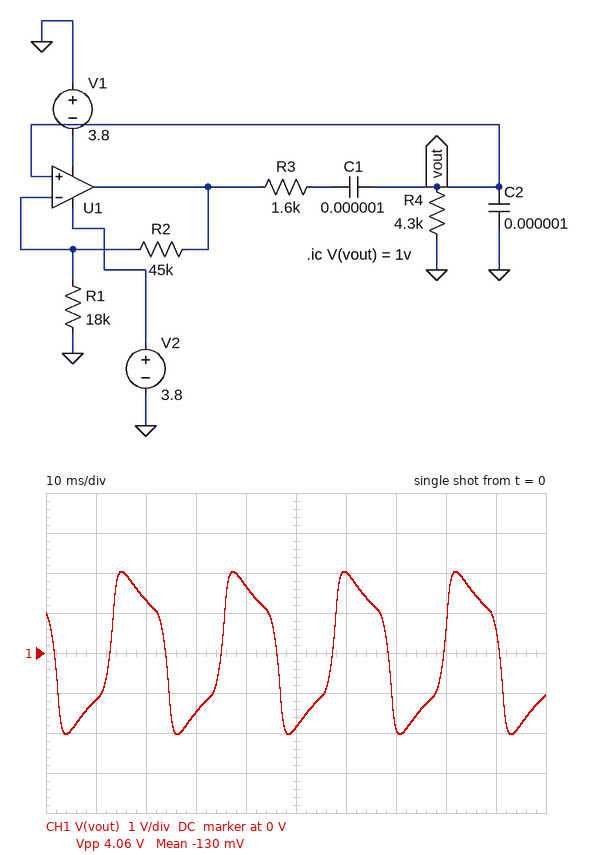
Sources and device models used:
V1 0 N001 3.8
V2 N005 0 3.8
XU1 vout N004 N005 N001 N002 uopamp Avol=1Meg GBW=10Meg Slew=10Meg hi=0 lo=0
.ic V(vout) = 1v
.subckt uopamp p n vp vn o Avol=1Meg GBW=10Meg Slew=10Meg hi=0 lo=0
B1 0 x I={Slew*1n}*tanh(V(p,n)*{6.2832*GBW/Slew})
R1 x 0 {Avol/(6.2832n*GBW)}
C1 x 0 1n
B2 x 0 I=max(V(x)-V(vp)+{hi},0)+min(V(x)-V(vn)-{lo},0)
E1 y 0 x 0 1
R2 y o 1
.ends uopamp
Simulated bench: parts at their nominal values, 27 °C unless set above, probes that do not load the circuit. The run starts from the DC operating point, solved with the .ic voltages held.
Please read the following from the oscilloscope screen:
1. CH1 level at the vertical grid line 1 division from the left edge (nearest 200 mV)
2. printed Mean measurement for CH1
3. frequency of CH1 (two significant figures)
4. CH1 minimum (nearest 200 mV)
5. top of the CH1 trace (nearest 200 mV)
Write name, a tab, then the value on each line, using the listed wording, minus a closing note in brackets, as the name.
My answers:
CH1 level at the vertical grid line 1 division from the left edge	-1.2 V
printed Mean measurement for CH1	-130 mV
frequency of CH1	45 Hz
CH1 minimum	-2.0 V
top of the CH1 trace	2.0 V
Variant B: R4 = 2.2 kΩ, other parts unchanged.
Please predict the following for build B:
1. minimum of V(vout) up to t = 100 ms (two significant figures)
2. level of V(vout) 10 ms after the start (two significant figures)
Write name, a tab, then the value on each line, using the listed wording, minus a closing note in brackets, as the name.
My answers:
minimum of V(vout) up to t = 100 ms	-1.7 V
level of V(vout) 10 ms after the start	1.7 V
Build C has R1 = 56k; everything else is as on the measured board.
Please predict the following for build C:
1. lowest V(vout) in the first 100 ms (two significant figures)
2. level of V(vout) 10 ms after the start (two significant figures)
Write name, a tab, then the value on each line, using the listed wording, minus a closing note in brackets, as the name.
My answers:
lowest V(vout) in the first 100 ms	-240 mV
level of V(vout) 10 ms after the start	-160 mV
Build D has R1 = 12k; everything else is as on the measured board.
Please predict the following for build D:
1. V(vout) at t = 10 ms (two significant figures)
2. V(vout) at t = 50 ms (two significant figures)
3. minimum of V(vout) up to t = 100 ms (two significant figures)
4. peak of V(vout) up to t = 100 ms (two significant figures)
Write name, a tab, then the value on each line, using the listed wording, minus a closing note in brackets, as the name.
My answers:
V(vout) at t = 10 ms	-1.4 V
V(vout) at t = 50 ms	1.8 V
minimum of V(vout) up to t = 100 ms	-2.2 V
peak of V(vout) up to t = 100 ms	2.2 V
